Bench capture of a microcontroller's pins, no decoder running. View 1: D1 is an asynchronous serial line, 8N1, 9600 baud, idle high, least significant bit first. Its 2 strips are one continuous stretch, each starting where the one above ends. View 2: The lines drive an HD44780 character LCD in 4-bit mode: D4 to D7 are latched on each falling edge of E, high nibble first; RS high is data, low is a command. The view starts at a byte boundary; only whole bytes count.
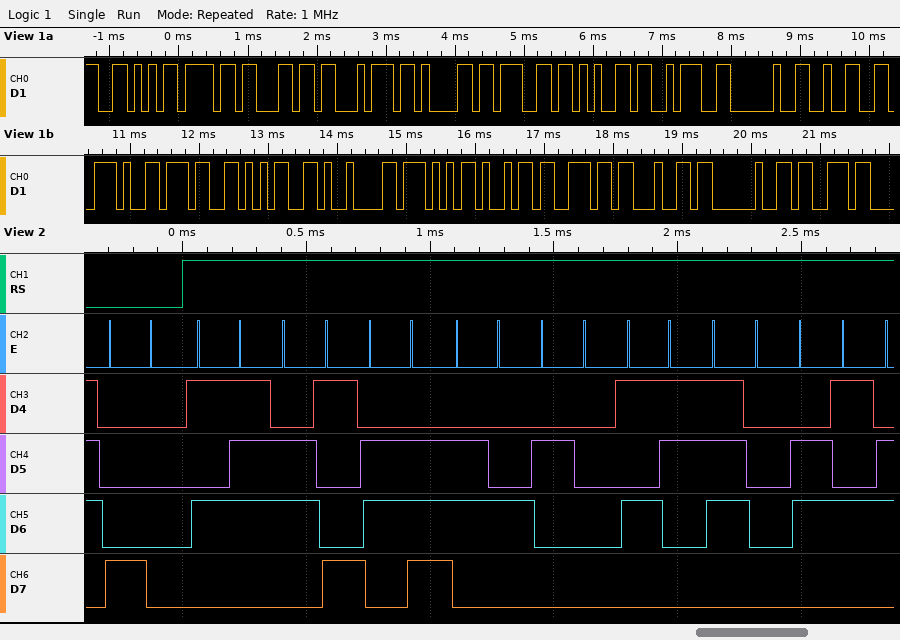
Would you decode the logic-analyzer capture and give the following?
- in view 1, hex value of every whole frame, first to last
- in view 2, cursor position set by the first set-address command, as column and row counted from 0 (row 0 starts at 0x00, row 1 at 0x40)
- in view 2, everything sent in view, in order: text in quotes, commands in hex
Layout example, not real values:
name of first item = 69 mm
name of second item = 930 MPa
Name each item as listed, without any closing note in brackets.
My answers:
in view 1, hex value of every whole frame, first to last = 56 6F 6C 74 61 67 65 3A 20 32 2E 37 35 09 57 69 6E 64 20 73
in view 2, cursor position set by the first set-address command, as column and row counted from 0 = column 0, row 0
in view 2, everything sent in view, in order: text in quotes, commands in hex = 0x80 "Wind Spe"
